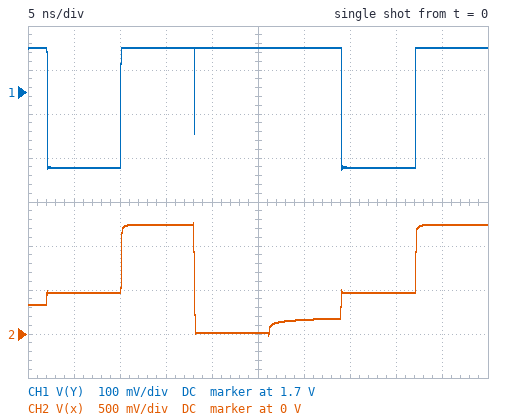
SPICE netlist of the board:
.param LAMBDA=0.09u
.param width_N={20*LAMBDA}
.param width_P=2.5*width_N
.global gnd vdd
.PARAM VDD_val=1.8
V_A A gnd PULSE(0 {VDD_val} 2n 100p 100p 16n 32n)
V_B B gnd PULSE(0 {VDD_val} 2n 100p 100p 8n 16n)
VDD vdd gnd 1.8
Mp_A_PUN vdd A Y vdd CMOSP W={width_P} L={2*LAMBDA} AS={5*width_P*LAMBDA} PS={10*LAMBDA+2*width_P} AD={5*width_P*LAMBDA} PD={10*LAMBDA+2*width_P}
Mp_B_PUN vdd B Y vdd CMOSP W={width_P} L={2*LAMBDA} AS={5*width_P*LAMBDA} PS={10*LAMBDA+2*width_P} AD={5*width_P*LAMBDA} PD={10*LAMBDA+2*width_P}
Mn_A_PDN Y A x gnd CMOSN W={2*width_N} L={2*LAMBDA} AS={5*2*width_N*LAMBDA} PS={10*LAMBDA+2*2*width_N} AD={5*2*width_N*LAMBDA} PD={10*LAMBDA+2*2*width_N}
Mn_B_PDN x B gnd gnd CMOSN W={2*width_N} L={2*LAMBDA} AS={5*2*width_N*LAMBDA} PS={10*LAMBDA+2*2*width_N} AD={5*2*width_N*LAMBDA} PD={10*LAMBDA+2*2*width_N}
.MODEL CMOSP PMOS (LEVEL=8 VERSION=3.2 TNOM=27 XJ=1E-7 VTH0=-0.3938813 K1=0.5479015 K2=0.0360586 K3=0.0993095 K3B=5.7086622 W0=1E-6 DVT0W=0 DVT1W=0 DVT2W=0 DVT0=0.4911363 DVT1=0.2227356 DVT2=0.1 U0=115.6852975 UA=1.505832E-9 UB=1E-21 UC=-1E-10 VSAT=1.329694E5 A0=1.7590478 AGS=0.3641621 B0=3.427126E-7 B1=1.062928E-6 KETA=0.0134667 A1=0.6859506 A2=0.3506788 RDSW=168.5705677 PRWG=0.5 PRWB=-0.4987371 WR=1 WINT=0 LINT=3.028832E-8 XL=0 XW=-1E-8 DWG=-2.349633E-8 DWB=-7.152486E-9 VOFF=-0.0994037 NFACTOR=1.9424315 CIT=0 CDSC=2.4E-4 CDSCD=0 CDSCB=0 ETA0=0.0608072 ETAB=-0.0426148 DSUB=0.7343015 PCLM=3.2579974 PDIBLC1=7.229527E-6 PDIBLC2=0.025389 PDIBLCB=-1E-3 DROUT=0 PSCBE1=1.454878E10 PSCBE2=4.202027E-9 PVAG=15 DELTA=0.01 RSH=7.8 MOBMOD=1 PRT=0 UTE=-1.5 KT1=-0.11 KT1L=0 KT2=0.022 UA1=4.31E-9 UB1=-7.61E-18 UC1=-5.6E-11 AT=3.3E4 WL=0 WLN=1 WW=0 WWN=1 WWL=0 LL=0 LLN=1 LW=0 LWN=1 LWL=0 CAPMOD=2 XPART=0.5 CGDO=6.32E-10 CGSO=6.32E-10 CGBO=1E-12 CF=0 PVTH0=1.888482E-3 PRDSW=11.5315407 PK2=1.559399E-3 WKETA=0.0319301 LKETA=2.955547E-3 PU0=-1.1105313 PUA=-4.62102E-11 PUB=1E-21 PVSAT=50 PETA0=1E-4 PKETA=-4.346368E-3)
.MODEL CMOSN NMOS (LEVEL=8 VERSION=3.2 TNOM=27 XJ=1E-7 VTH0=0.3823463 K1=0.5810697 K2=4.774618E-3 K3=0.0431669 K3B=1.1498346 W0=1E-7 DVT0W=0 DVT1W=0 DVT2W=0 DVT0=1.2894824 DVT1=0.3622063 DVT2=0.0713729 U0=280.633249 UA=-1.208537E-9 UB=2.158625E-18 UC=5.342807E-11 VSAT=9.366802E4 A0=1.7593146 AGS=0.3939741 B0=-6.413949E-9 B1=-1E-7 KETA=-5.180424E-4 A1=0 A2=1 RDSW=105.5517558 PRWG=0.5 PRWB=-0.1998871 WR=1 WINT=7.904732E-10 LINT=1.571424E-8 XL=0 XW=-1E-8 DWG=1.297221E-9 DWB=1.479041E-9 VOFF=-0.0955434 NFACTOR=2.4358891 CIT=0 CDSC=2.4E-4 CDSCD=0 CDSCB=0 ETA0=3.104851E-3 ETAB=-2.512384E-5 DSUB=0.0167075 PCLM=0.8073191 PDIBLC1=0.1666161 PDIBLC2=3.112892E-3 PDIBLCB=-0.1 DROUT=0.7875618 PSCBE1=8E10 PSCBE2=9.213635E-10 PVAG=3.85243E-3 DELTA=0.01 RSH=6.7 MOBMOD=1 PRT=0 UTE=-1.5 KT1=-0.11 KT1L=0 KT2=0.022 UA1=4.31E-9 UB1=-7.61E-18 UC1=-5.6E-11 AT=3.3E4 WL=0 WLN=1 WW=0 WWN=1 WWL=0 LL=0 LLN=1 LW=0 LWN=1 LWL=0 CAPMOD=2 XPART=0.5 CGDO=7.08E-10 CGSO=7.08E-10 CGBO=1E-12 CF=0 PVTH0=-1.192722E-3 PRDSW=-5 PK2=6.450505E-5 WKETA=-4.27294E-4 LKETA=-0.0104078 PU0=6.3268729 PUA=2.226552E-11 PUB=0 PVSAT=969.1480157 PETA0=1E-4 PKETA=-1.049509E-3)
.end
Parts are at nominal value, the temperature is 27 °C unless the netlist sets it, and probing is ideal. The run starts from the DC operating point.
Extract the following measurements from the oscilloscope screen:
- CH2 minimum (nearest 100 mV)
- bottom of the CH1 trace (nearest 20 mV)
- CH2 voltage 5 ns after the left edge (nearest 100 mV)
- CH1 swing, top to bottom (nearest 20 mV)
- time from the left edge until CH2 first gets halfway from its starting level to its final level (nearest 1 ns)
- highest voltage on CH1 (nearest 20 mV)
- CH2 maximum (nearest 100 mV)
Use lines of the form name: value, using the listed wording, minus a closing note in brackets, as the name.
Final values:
CH2 minimum: 0 V
bottom of the CH1 trace: 1.52 V
CH2 voltage 5 ns after the left edge: 500 mV
CH1 swing, top to bottom: 280 mV
time from the left edge until CH2 first gets halfway from its starting level to its final level: 10 ns
highest voltage on CH1: 1.80 V
CH2 maximum: 1.3 V
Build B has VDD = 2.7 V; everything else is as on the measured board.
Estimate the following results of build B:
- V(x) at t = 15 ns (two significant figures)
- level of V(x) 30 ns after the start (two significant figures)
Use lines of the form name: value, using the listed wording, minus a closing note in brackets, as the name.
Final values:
V(x) at t = 15 ns: 1.4 V
level of V(x) 30 ns after the start: 370 mV
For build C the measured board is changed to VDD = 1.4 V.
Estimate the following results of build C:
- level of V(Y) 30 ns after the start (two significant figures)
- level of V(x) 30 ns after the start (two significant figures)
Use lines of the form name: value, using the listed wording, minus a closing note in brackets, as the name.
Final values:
level of V(Y) 30 ns after the start: 1.4 V
level of V(x) 30 ns after the start: 68 mV
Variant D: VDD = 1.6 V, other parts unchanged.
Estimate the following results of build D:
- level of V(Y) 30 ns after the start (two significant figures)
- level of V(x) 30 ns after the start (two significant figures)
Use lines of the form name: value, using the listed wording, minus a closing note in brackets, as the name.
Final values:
level of V(Y) 30 ns after the start: 1.6 V
level of V(x) 30 ns after the start: 110 mV
